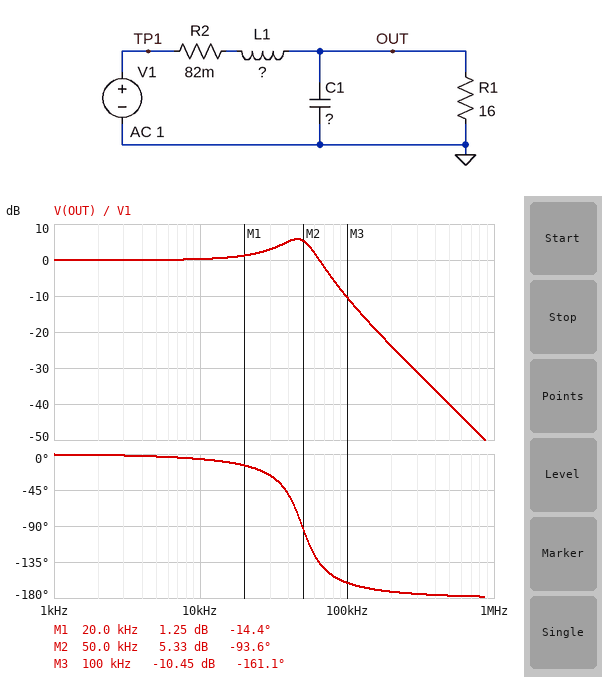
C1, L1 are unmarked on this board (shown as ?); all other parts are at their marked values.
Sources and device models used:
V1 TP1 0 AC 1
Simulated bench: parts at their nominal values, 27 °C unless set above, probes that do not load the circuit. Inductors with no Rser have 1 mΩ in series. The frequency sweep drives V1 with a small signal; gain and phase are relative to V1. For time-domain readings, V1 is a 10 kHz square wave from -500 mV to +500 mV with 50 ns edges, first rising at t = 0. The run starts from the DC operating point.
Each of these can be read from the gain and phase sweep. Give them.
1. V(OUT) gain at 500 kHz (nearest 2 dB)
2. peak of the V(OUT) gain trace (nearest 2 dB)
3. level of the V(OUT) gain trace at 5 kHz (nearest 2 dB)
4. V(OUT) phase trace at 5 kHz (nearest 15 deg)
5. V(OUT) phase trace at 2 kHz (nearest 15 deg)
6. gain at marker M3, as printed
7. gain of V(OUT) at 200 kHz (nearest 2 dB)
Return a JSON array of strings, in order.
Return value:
["-40 dB", "6 dB", "0 dB", "0 deg", "0 deg", "-10.45 dB", "-24 dB"]
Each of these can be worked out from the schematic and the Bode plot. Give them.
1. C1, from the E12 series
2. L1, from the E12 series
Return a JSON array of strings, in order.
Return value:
["390 nF", "27 µH"]
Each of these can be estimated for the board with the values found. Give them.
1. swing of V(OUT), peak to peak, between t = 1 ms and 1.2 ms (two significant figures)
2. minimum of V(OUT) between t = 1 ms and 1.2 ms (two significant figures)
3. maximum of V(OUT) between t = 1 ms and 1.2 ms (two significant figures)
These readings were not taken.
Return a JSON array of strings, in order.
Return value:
["1.8 V", "-920 mV", "920 mV"]
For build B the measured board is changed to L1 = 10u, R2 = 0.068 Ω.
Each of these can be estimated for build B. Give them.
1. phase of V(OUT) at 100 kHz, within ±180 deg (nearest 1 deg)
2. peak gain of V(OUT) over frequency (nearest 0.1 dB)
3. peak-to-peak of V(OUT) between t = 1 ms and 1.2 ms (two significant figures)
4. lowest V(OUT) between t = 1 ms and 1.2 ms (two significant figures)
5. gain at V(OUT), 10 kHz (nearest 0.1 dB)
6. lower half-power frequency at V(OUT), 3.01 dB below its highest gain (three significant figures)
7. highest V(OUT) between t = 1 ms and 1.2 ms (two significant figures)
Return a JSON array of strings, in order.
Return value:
["-143 deg", "9.7 dB", "2.2 V", "-1.1 V", "0.1 dB", "63.6 kHz", "1.1 V"]
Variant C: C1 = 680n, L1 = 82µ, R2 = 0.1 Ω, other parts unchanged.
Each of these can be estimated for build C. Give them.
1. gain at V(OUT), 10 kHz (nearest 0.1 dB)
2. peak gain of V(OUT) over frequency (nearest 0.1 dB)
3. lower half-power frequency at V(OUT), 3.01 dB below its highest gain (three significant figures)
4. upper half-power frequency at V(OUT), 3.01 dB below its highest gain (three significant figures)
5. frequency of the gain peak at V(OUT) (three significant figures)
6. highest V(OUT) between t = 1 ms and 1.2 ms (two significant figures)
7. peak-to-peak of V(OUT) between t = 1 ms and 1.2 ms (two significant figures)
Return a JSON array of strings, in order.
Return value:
["1.4 dB", "3.7 dB", "7.07 kHz", "25.4 kHz", "18.6 kHz", "780 mV", "1.6 V"]
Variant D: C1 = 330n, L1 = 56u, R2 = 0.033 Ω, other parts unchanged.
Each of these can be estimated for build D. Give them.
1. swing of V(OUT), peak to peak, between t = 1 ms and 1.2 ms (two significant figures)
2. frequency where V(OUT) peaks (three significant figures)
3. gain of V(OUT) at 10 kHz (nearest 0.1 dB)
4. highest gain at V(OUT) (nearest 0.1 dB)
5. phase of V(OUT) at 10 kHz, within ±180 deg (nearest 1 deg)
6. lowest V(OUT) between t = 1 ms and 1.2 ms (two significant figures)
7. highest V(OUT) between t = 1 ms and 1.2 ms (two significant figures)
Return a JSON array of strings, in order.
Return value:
["1.5 V", "30.3 kHz", "0.4 dB", "2.5 dB", "-13 deg", "-750 mV", "750 mV"]
